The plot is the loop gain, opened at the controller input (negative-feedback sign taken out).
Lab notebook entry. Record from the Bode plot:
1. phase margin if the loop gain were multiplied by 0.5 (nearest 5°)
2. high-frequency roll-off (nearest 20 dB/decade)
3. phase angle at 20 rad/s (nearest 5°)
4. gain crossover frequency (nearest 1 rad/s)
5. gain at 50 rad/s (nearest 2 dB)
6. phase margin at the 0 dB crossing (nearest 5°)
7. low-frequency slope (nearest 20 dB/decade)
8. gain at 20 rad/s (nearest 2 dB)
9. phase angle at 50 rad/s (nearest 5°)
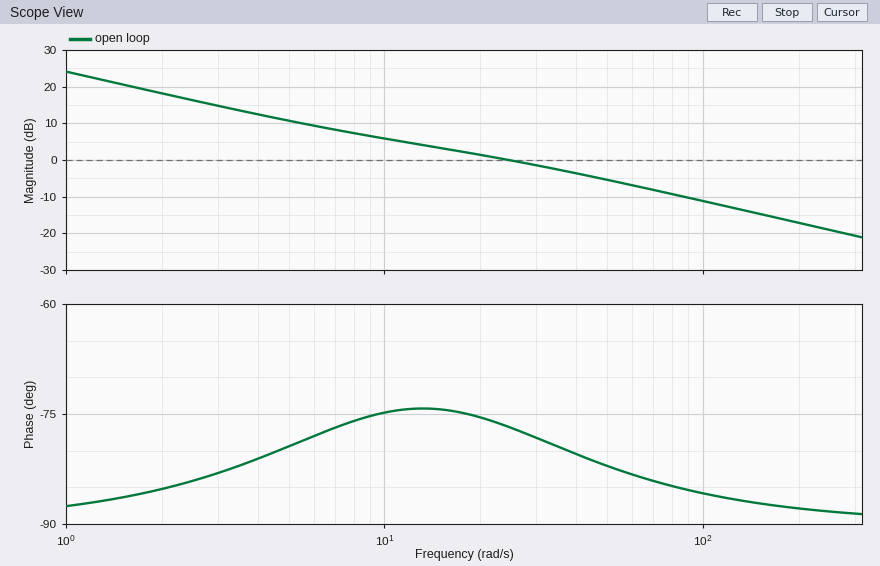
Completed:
105°
-20 dB/decade
-75°
25 rad/s
-6 dB
105°
-20 dB/decade
2 dB
-80°
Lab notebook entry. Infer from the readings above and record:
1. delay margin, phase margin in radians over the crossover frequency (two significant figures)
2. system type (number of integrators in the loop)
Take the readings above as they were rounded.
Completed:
0.073 s
1
